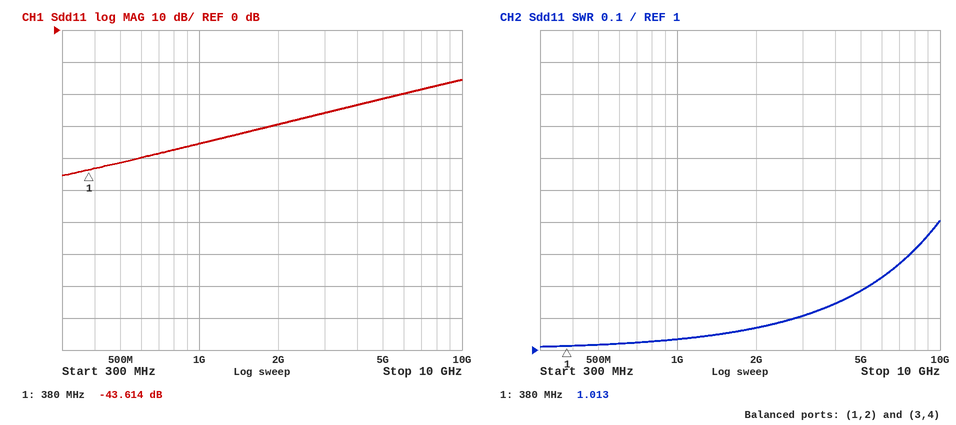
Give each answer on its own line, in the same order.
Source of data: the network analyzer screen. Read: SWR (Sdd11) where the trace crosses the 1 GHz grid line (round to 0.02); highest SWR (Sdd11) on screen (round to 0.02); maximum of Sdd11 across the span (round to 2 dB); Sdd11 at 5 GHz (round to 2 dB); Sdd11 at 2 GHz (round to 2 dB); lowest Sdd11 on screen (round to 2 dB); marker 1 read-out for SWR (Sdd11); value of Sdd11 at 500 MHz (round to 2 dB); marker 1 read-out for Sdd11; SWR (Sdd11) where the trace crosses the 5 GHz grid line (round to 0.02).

1.04
1.40
-16 dB
-22 dB
-30 dB
-46 dB
1.013
-42 dB
-43.614 dB
1.18
